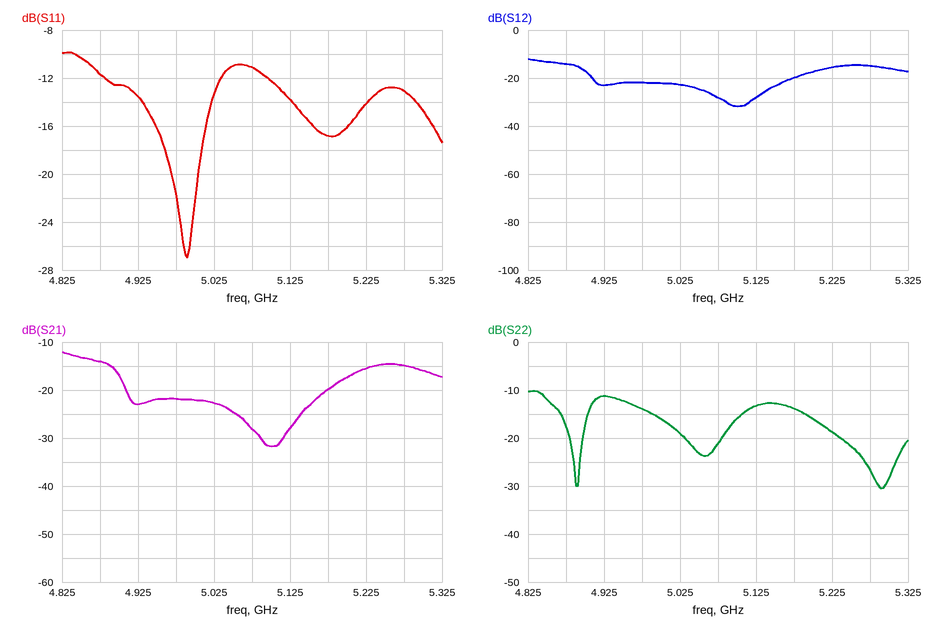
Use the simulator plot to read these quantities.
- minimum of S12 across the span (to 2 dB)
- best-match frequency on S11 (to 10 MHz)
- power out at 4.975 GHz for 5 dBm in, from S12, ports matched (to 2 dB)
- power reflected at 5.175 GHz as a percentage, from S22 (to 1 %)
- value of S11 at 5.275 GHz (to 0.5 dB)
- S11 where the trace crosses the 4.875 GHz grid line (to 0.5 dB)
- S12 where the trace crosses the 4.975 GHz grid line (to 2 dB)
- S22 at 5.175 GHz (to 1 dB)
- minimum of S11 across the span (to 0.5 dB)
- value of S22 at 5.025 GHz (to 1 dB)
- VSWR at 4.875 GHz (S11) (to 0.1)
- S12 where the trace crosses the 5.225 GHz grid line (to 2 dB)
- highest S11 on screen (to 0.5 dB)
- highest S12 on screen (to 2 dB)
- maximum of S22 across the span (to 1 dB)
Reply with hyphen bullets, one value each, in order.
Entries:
- -32 dB
- 4.99 GHz
- -16 dBm
- 4 %
- -13.0 dB
- -11.5 dB
- -22 dB
- -14 dB
- -27.0 dB
- -19 dB
- 1.7
- -16 dB
- -10.0 dB
- -12 dB
- -10 dB
